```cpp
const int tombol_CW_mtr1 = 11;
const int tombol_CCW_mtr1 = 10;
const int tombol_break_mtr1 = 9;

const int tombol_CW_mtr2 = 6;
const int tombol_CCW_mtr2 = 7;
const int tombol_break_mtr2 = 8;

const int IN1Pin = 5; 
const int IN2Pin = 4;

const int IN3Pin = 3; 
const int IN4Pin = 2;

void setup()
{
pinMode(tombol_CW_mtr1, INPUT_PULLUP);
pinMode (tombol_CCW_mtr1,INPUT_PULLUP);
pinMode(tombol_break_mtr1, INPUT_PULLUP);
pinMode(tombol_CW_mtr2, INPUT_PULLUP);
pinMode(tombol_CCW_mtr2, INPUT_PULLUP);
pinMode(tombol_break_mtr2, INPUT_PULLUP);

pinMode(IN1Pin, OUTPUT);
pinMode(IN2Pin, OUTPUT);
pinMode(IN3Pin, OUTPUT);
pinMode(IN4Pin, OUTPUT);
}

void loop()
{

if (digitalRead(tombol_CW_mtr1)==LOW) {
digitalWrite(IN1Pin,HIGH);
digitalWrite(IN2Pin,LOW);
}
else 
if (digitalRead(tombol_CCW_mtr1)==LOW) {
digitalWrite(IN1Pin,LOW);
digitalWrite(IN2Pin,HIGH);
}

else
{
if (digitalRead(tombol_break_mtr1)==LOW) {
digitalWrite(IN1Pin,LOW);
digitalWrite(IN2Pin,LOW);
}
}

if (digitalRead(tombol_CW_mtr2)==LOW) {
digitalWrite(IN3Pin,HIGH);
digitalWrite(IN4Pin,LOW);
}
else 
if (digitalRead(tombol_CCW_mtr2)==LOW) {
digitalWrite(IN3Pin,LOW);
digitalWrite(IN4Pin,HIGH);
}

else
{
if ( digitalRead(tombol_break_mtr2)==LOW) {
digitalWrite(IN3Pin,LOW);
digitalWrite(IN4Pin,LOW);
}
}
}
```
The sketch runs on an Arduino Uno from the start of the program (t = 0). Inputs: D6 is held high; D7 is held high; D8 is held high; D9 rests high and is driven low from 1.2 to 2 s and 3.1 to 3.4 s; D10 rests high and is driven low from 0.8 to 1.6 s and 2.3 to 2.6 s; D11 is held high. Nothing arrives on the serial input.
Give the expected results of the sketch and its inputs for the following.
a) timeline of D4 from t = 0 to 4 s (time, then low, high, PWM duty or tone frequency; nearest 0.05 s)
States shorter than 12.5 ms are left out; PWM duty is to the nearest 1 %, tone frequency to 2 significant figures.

0 s low; 0.8 s high; 1.6 s low; 2.3 s high; 3.1 s low
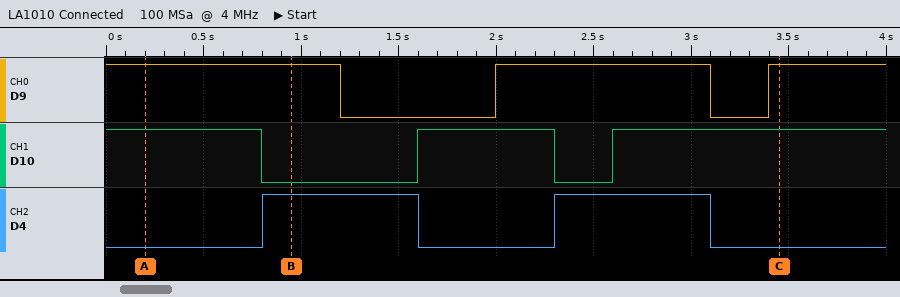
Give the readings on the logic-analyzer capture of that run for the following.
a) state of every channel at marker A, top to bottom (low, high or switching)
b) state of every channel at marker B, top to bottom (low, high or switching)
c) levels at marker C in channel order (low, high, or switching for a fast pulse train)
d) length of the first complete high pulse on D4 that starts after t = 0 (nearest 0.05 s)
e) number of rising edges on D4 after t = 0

D9 high, D10 high, D4 low
D9 high, D10 low, D4 high
D9 high, D10 high, D4 low
0.80 s
2
